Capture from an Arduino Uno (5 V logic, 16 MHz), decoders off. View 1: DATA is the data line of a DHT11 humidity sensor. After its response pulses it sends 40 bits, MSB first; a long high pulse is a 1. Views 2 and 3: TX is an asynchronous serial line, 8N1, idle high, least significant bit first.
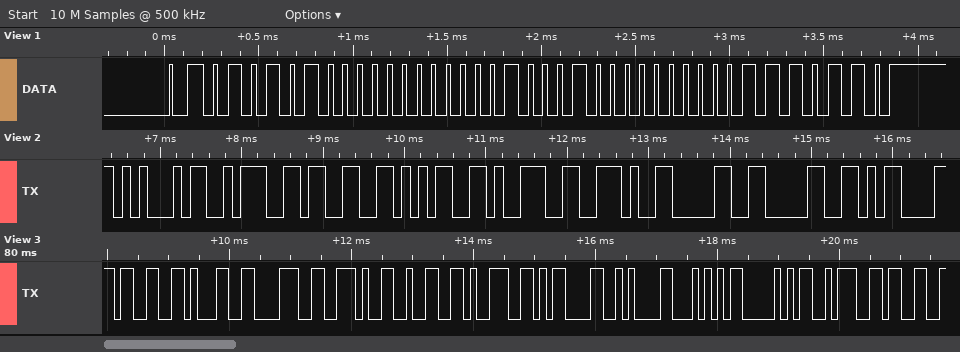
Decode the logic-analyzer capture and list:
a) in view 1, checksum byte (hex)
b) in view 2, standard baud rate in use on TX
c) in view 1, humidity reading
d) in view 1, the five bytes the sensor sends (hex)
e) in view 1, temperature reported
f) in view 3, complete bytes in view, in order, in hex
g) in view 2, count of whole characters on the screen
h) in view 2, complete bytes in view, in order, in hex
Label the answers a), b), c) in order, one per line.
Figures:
a) 0x76
b) 9600 baud
c) 84 %
d) 54 00 22 00 76
e) 34.0 °C
f) 33 31 38 2E 32 39 0D 0A 54 50 3A 33
g) 9
h) 45 3A 33 35 39 2E 30 30 0D
